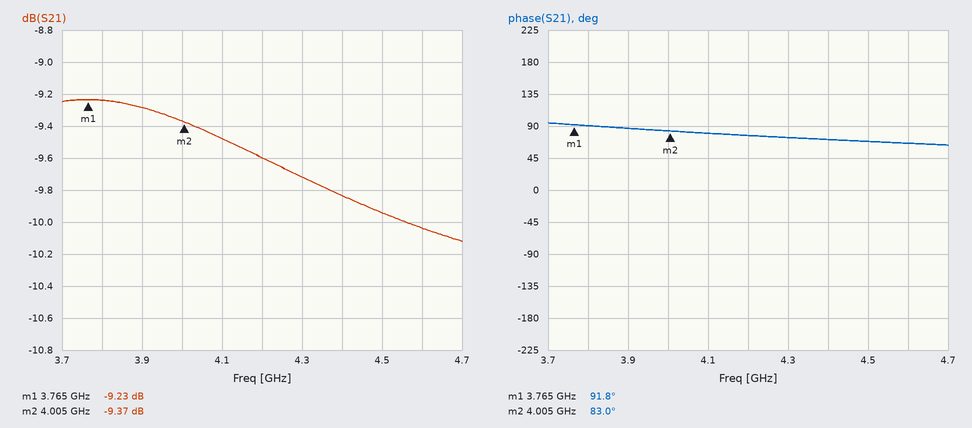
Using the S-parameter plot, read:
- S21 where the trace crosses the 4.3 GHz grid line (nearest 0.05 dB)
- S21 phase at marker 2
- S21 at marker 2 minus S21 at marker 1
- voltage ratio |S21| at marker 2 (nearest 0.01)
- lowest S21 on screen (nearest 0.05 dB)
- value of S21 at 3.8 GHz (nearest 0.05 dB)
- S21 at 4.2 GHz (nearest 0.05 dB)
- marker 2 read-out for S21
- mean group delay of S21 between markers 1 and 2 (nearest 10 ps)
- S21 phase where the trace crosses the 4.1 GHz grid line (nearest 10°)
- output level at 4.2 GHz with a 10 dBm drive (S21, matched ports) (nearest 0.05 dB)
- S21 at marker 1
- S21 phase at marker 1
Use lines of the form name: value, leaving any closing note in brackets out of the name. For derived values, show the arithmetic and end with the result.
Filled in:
S21 where the trace crosses the 4.3 GHz grid line: -9.70 dB
S21 phase at marker 2: 83.0°
S21 at marker 2 minus S21 at marker 1: -9.37 − (-9.23) = -0.14 dB
voltage ratio |S21| at marker 2: 10^(-9.37/20) ≈ 0.34
lowest S21 on screen: -10.10 dB
value of S21 at 3.8 GHz: -9.25 dB
S21 at 4.2 GHz: -9.60 dB
marker 2 read-out for S21: -9.37 dB
mean group delay of S21 between markers 1 and 2: −(83° − (91.8°))/(360° × 240 MHz) ≈ 102 ps, so 100 ps to the nearest 10 ps
S21 phase where the trace crosses the 4.1 GHz grid line: 80°
output level at 4.2 GHz with a 10 dBm drive (S21, matched ports): 10 dBm + (-9.60 dB) = 0.40 dBm
S21 at marker 1: -9.23 dB
S21 phase at marker 1: 91.8°
